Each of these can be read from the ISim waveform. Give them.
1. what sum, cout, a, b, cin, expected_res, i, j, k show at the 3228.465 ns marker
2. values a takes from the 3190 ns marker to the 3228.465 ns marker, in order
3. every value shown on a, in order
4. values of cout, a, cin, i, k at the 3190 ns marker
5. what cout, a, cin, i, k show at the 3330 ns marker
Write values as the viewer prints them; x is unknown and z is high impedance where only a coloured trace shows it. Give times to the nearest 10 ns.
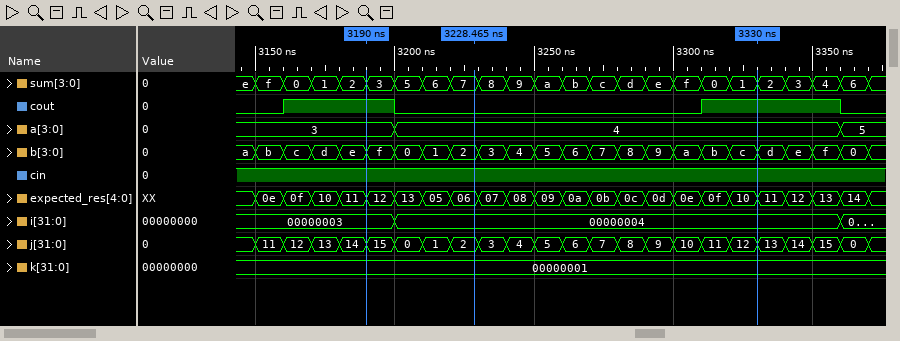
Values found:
sum=7, cout=0, a=4, b=2, cin=1, expected_res=06, i=00000004, j=2, k=00000001
3, 4
3, 4, 5
cout=1, a=3, cin=1, i=00000003, k=00000001
cout=1, a=4, cin=1, i=00000004, k=00000001
